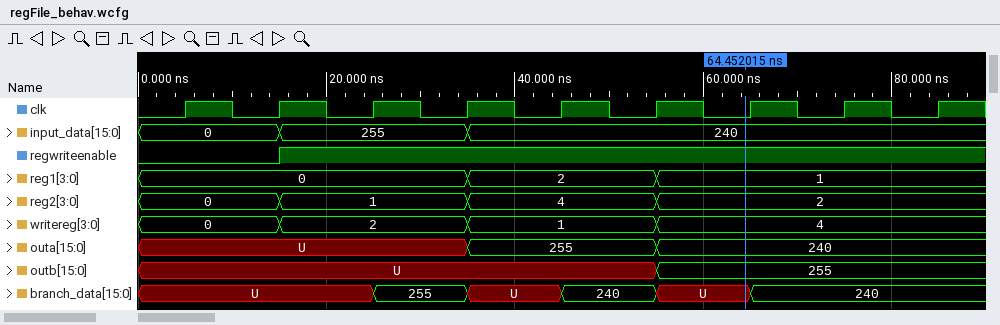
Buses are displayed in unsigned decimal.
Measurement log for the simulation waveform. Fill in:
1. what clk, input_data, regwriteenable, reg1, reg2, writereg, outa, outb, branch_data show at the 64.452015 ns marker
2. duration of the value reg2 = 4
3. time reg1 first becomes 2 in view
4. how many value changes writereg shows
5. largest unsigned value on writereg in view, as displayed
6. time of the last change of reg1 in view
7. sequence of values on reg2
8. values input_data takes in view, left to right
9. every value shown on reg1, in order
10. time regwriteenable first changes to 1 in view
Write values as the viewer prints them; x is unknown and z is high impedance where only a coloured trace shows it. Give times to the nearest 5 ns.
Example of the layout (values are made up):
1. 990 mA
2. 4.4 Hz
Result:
1. clk=0, input_data=240, regwriteenable=1, reg1=1, reg2=2, writereg=4, outa=240, outb=255, branch_data=U
2. 20 ns
3. 35 ns
4. 3
5. 4
6. 55 ns
7. 0, 1, 4, 2
8. 0, 255, 240
9. 0, 2, 1
10. 15 ns
